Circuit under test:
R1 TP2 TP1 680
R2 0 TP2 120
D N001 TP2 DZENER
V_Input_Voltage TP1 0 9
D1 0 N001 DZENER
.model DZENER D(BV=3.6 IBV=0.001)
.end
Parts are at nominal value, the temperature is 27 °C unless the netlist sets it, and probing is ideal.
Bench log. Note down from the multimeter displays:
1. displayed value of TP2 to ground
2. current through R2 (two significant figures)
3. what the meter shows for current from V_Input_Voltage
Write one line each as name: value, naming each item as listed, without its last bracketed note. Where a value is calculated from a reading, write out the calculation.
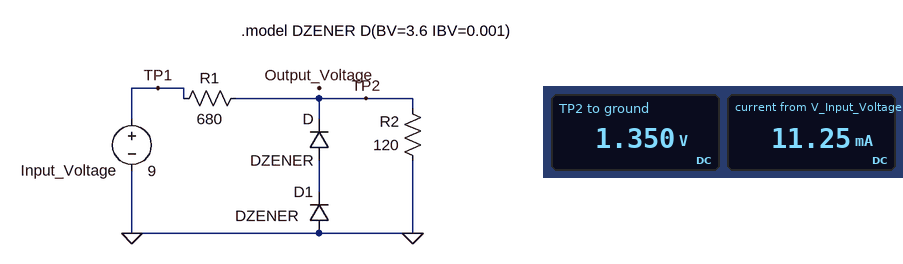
displayed value of TP2 to ground: 1.350 V
current through R2: (1.35 V) / 120 Ω = 11 mA
what the meter shows for current from V_Input_Voltage: 11.25 mA
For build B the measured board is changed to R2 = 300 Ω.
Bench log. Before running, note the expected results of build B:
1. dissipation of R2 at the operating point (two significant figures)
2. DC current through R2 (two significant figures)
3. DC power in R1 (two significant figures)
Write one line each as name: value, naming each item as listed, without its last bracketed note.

dissipation of R2 at the operating point: 25 mW
DC current through R2: 9.2 mA
DC power in R1: 57 mW
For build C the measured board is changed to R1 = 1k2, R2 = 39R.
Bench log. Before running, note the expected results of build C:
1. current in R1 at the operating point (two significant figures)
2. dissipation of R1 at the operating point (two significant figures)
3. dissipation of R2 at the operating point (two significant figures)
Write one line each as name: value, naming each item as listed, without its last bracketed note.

current in R1 at the operating point: 7.3 mA
dissipation of R1 at the operating point: 63 mW
dissipation of R2 at the operating point: 2.1 mW
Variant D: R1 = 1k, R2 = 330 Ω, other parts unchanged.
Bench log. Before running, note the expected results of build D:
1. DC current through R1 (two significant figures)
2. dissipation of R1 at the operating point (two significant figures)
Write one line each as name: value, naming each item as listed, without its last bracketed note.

DC current through R1: 6.8 mA
dissipation of R1 at the operating point: 46 mW
